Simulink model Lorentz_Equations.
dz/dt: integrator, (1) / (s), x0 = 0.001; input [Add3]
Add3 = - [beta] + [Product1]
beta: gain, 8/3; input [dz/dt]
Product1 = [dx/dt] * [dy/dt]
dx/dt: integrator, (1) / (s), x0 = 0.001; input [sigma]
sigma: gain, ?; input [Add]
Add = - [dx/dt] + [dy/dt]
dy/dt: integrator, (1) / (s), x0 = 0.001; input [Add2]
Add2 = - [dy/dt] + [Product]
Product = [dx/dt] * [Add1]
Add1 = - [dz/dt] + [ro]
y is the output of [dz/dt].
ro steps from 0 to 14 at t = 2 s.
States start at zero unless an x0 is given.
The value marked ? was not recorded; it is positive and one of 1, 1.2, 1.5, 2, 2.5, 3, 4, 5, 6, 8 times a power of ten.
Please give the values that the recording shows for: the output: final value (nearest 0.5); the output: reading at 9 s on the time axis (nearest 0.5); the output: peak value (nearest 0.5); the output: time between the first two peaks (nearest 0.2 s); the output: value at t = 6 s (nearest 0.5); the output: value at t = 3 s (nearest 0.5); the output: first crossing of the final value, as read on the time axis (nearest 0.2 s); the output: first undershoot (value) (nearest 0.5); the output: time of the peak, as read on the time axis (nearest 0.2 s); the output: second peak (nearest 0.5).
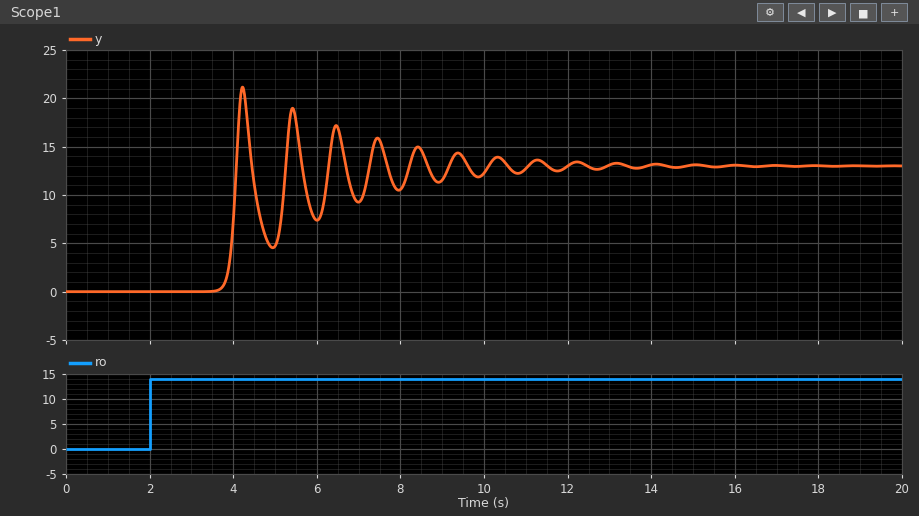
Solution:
13.0
11.5
21.0
1.2 s
7.5
0.0
4.0 s
4.5
4.2 s
19.0
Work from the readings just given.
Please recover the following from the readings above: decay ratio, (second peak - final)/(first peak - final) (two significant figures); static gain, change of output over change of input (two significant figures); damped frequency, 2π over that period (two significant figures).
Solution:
0.75
0.93
5.2 rad/s
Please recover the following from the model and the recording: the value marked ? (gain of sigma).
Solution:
5
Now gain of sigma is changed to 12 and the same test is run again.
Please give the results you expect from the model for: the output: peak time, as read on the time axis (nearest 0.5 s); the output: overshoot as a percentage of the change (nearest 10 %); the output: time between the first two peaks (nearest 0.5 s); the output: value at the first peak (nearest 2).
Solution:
3.5 s
70 %
1.5 s
22
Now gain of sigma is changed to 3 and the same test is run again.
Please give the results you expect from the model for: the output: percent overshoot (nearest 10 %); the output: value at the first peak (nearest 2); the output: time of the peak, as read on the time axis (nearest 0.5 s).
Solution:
60 %
20
4.5 s
